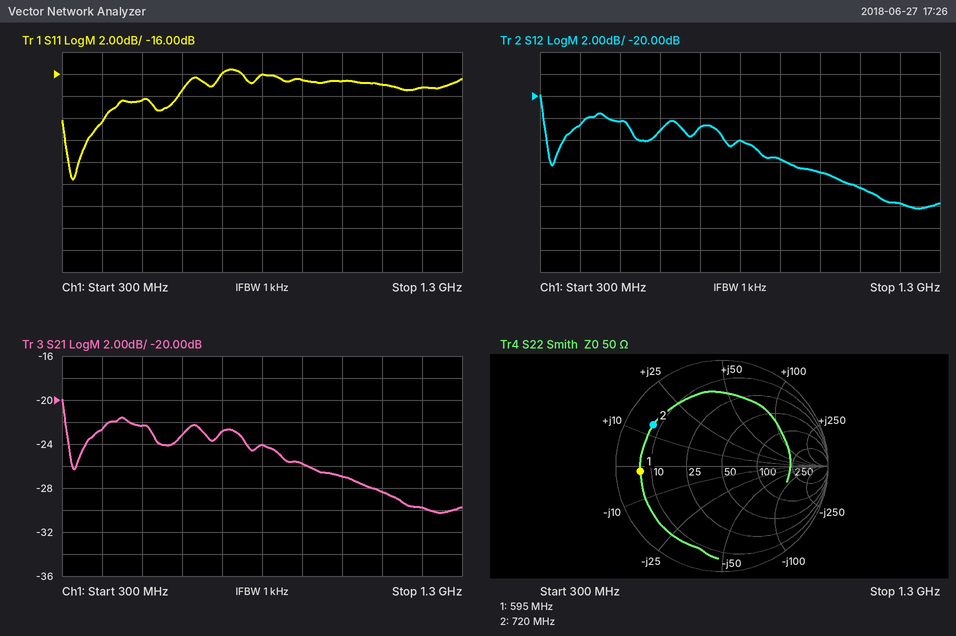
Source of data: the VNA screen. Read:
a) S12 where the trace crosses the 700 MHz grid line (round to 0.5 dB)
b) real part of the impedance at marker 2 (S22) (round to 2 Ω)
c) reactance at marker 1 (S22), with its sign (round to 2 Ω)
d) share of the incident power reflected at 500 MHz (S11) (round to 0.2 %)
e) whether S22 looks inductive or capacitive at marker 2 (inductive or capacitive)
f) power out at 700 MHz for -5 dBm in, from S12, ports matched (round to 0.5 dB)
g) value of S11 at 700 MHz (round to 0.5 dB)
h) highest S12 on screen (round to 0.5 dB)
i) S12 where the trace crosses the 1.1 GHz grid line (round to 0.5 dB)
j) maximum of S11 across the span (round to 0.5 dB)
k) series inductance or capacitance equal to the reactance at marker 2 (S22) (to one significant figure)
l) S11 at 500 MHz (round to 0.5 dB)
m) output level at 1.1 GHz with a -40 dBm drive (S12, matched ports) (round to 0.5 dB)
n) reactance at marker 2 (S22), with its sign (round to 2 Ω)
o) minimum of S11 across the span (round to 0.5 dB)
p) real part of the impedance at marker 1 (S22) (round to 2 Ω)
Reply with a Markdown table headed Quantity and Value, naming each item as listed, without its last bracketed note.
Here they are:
| Quantity | Value |
|---|---|
| S12 where the trace crosses the 700 MHz grid line | -23.0 dB |
| real part of the impedance at marker 2 (S22) | 8 Ω |
| reactance at marker 1 (S22), with its sign | -2 Ω |
| share of the incident power reflected at 500 MHz (S11) | 1.4 % |
| whether S22 looks inductive or capacitive at marker 2 | inductive |
| power out at 700 MHz for -5 dBm in, from S12, ports matched | -28.0 dBm |
| value of S11 at 700 MHz | -16.0 dB |
| highest S12 on screen | -20.0 dB |
| S12 where the trace crosses the 1.1 GHz grid line | -28.5 dB |
| maximum of S11 across the span | -15.5 dB |
| series inductance or capacitance equal to the reactance at marker 2 (S22) | 3 nH |
| S11 at 500 MHz | -18.5 dB |
| output level at 1.1 GHz with a -40 dBm drive (S12, matched ports) | -68.5 dBm |
| reactance at marker 2 (S22), with its sign | +14 Ω |
| minimum of S11 across the span | -25.5 dB |
| real part of the impedance at marker 1 (S22) | 6 Ω |
